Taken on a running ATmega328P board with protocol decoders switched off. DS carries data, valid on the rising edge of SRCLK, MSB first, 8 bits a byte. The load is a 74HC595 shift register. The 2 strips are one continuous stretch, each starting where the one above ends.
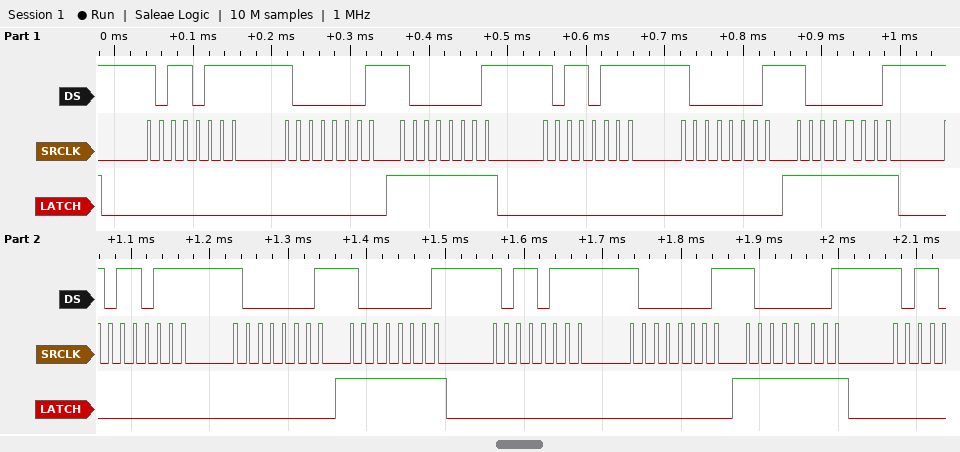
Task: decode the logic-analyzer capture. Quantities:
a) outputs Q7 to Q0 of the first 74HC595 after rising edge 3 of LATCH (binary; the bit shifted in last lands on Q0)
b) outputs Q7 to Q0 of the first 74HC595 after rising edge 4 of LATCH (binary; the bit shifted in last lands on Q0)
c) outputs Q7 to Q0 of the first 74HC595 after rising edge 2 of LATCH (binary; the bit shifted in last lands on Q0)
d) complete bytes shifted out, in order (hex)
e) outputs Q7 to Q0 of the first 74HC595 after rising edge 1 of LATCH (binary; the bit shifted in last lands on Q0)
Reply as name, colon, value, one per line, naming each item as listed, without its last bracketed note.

outputs Q7 to Q0 of the first 74HC595 after rising edge 3 of LATCH: 10000001
outputs Q7 to Q0 of the first 74HC595 after rising edge 4 of LATCH: 10000001
outputs Q7 to Q0 of the first 74HC595 after rising edge 2 of LATCH: 10000001
complete bytes shifted out, in order: B7 81 81 B7 81 81 B7 81 81 B7 81 81
outputs Q7 to Q0 of the first 74HC595 after rising edge 1 of LATCH: 10000001
